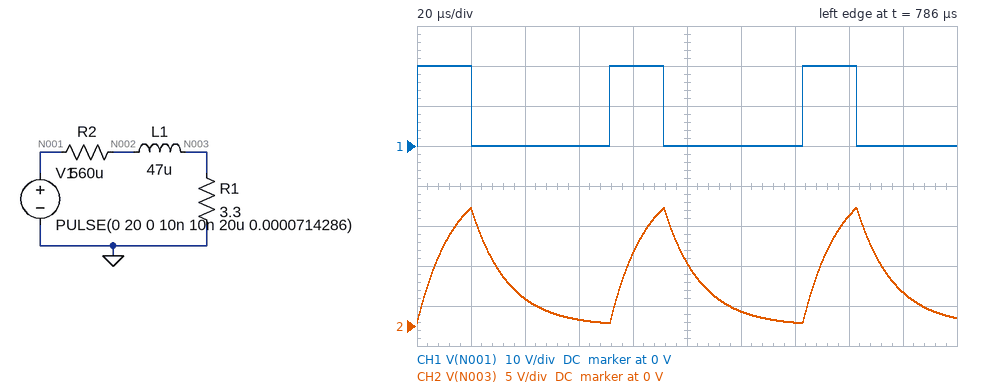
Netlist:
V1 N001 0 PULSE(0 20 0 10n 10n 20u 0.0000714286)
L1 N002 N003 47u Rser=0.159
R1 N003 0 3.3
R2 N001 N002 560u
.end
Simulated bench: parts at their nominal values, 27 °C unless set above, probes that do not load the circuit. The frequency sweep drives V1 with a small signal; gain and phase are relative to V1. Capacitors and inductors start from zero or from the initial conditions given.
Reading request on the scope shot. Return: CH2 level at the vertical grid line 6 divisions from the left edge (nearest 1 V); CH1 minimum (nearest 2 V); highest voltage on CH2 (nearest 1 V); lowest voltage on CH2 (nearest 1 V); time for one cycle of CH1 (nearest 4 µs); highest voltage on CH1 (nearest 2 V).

2 V
0 V
15 V
0 V
72 µs
20 V
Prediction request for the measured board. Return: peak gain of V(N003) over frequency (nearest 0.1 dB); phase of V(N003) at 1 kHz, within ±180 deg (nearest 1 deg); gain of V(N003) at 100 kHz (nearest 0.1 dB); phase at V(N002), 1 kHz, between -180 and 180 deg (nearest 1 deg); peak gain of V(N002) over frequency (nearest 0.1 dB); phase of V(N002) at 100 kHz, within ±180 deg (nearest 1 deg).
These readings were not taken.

-0.4 dB
-5 deg
-19.1 dB
0 deg
0 dB
0 deg
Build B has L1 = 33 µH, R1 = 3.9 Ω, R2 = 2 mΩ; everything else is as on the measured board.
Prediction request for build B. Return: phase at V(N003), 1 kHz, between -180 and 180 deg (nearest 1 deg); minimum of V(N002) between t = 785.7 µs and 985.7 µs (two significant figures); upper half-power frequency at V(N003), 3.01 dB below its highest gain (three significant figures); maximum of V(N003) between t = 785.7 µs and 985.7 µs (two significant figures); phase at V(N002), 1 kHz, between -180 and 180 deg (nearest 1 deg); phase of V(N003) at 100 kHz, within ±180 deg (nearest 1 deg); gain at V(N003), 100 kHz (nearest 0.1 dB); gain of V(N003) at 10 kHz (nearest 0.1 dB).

-3 deg
-9.0 mV
19.6 kHz
18 V
0 deg
-79 deg
-14.7 dB
-1.4 dB
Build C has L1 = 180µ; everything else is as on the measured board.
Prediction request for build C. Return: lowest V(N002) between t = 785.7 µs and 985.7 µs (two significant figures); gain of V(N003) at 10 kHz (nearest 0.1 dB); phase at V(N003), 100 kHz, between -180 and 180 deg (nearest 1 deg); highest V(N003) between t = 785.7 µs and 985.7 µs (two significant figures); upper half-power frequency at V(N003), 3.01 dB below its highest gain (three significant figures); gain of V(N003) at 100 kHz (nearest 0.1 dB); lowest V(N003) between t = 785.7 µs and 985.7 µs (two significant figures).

-1.4 mV
-11.1 dB
-88 deg
8.2 V
3.06 kHz
-30.7 dB
3.0 V
